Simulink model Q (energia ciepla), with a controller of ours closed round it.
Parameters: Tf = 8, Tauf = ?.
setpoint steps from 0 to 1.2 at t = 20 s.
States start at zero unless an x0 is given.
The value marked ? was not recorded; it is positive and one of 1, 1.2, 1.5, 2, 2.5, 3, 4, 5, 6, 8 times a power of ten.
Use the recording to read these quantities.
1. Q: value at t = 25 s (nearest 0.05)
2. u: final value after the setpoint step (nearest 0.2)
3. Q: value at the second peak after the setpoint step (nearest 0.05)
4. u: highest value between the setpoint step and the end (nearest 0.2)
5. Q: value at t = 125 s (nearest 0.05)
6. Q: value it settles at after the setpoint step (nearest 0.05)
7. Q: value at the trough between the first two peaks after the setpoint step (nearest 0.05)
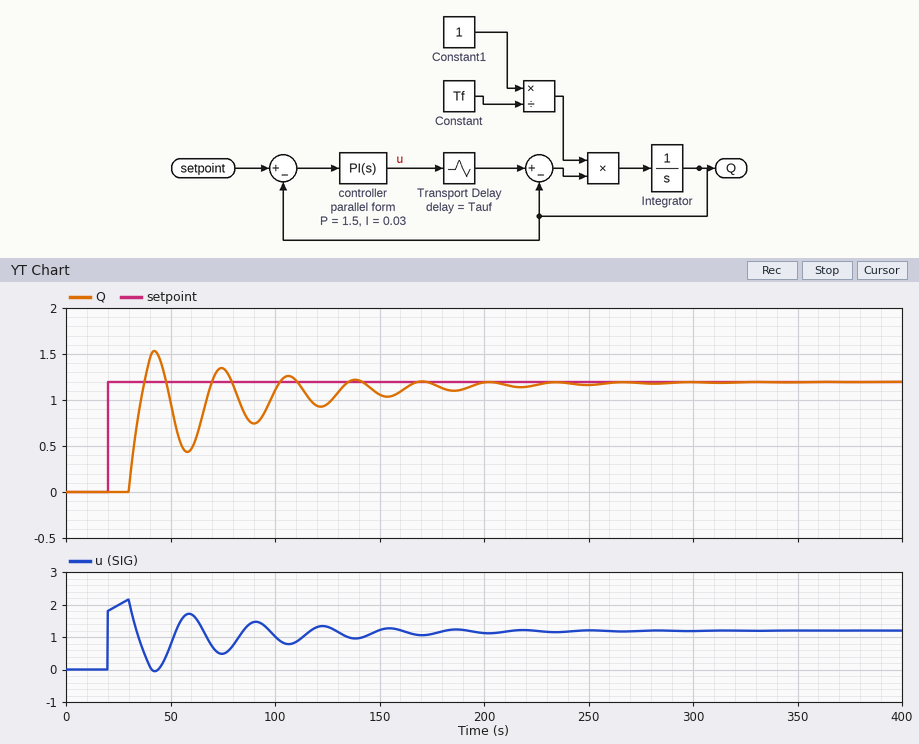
0.00
1.2
1.35
2.2
0.95
1.20
0.45
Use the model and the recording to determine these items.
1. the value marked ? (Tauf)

10
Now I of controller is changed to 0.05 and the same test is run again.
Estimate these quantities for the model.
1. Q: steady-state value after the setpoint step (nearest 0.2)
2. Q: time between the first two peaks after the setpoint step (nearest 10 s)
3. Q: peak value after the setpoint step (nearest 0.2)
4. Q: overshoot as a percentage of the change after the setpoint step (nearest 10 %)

1.2
30 s
1.6
40 %
